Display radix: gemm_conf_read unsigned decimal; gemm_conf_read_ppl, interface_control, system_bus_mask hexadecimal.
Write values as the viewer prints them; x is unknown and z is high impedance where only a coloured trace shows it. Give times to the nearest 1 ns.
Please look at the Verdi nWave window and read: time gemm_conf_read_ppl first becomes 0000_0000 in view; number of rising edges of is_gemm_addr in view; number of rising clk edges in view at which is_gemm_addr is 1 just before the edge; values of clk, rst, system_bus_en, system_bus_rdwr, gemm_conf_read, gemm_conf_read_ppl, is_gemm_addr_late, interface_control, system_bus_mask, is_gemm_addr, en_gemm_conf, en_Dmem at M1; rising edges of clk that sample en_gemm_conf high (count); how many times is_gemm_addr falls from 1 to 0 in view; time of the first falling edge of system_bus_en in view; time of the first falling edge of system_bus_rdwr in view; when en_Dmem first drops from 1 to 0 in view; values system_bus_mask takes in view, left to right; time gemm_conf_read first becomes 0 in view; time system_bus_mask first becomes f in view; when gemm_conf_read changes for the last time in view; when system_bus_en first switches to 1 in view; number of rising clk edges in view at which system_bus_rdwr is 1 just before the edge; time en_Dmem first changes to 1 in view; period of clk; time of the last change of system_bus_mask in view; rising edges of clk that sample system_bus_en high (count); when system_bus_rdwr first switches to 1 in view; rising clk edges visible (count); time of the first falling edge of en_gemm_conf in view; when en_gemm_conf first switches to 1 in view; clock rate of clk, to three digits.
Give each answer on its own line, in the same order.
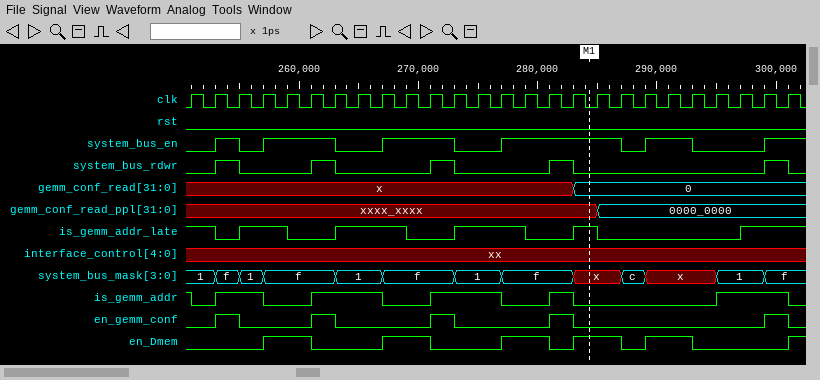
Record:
285 ns
5
13
clk=0, rst=0, system_bus_en=1, system_bus_rdwr=0, gemm_conf_read=0, gemm_conf_read_ppl=xxxx_xxxx, is_gemm_addr_late=1, interface_control=xx, system_bus_mask=x, is_gemm_addr=0, en_gemm_conf=0, en_Dmem=1
5
6
255 ns
255 ns
261 ns
1, f, 1, f, 1, f, 1, f, x, c, x, 1, f
283 ns
253 ns
283 ns
253 ns
5
257 ns
2 ns
299 ns
15
253 ns
26
255 ns
253 ns
500 MHz
